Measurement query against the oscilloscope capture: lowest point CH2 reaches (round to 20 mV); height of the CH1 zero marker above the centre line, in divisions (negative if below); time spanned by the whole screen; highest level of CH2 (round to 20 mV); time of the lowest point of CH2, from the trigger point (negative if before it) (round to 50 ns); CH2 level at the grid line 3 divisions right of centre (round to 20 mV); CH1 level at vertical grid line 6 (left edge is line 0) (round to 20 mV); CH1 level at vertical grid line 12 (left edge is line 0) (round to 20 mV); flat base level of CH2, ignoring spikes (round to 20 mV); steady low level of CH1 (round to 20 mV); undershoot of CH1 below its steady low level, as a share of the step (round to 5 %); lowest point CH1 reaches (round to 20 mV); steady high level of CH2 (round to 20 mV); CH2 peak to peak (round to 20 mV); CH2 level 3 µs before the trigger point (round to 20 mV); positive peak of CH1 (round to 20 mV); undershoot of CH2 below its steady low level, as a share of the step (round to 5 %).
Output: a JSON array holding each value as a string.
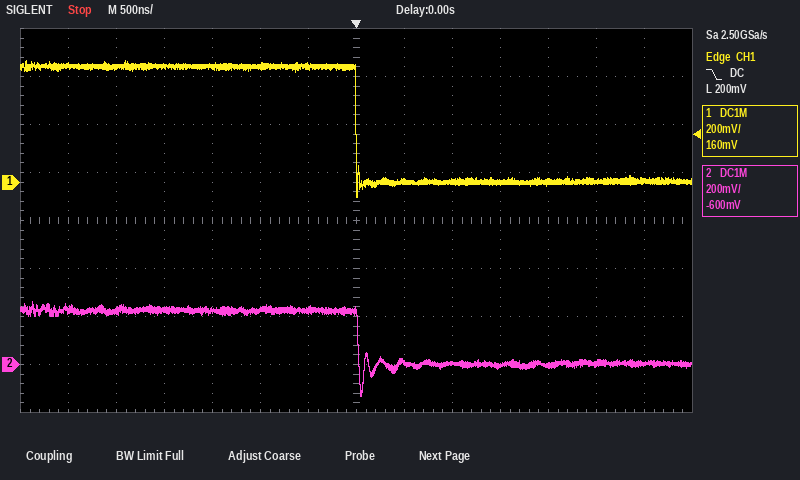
["-140 mV", "+0.8 div", "7 µs", "260 mV", "+50 ns", "0 mV", "480 mV", "0 mV", "0 mV", "0 mV", "15 %", "-60 mV", "220 mV", "400 mV", "220 mV", "500 mV", "60 %"]
